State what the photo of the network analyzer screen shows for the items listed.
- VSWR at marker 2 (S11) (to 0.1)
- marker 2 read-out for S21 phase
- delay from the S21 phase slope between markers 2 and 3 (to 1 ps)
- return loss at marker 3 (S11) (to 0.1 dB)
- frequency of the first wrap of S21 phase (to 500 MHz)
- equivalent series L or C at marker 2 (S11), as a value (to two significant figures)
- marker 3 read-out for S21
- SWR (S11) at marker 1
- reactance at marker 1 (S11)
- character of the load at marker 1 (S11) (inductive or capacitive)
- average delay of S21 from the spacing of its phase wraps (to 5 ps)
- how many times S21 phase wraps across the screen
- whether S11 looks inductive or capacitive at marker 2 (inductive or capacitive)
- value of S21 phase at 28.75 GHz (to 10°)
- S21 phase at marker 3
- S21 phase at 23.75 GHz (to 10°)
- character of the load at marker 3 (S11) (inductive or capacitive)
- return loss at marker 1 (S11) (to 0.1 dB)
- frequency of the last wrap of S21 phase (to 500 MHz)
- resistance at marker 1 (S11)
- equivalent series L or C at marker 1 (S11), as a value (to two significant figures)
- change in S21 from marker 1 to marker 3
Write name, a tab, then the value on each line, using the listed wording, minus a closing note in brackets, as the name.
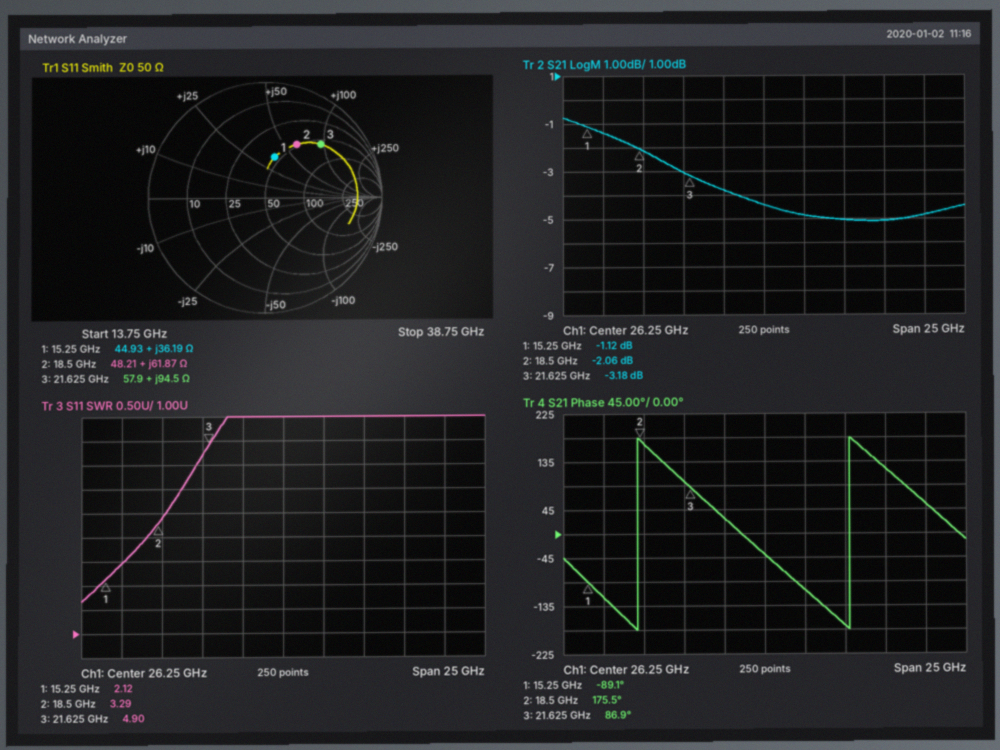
VSWR at marker 2 (S11)	3.3
marker 2 read-out for S21 phase	175.5°
delay from the S21 phase slope between markers 2 and 3	79 ps
return loss at marker 3 (S11)	3.6 dB
frequency of the first wrap of S21 phase	18.5 GHz
equivalent series L or C at marker 2 (S11), as a value	530 pH
marker 3 read-out for S21	-3.18 dB
SWR (S11) at marker 1	2.12
reactance at marker 1	+36.19 Ω
character of the load at marker 1 (S11)	inductive
average delay of S21 from the spacing of its phase wraps	75 ps
how many times S21 phase wraps across the screen	2
whether S11 looks inductive or capacitive at marker 2	inductive
value of S21 phase at 28.75 GHz	-110°
S21 phase at marker 3	86.9°
S21 phase at 23.75 GHz	30°
character of the load at marker 3 (S11)	inductive
return loss at marker 1 (S11)	8.9 dB
frequency of the last wrap of S21 phase	31.5 GHz
resistance at marker 1	44.93 Ω
equivalent series L or C at marker 1 (S11), as a value	380 pH
change in S21 from marker 1 to marker 3	-2.06 dB
